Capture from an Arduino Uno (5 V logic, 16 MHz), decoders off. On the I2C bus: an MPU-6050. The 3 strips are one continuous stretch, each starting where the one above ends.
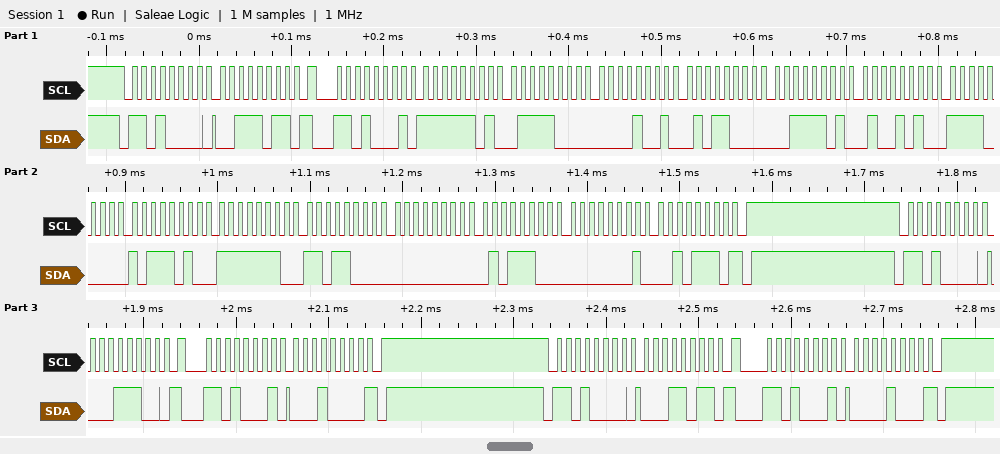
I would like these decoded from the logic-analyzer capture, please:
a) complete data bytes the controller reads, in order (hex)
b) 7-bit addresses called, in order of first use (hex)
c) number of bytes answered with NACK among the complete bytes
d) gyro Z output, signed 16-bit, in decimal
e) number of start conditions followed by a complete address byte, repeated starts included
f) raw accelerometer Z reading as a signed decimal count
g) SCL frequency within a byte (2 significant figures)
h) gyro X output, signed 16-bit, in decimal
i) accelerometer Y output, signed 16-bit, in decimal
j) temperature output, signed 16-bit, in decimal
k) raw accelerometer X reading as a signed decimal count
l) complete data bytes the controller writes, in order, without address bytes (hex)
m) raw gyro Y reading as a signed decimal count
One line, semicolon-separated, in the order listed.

FD 78 09 58 3D 4A F0 BA FE D8 00 5C 01 2E 10 08; 0x68; 3; 302; 6; 15690; 100 kHz; -296; 2392; -3910; -648; 3B 1C 1B; 92
